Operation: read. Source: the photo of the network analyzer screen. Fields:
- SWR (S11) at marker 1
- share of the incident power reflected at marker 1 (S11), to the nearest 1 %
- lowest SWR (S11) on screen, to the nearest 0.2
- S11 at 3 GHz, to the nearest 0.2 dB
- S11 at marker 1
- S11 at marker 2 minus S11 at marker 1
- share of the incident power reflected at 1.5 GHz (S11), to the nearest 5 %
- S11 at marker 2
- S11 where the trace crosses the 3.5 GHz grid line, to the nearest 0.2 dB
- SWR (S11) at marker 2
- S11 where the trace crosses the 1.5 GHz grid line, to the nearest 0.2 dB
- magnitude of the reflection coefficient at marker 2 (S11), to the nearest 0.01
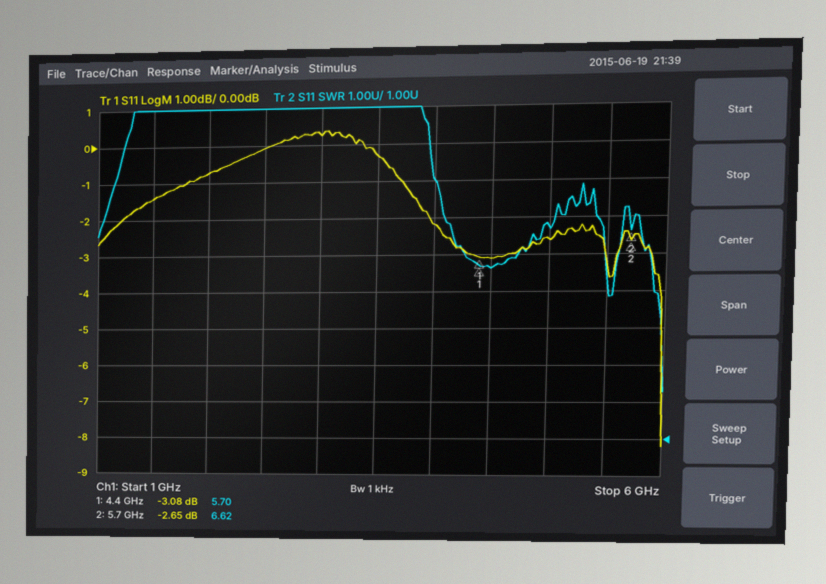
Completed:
5.70
49 %
2.2
0.2 dB
-3.08 dB
0.43 dB
70 %
-2.65 dB
-0.4 dB
6.62
-1.4 dB
0.74
